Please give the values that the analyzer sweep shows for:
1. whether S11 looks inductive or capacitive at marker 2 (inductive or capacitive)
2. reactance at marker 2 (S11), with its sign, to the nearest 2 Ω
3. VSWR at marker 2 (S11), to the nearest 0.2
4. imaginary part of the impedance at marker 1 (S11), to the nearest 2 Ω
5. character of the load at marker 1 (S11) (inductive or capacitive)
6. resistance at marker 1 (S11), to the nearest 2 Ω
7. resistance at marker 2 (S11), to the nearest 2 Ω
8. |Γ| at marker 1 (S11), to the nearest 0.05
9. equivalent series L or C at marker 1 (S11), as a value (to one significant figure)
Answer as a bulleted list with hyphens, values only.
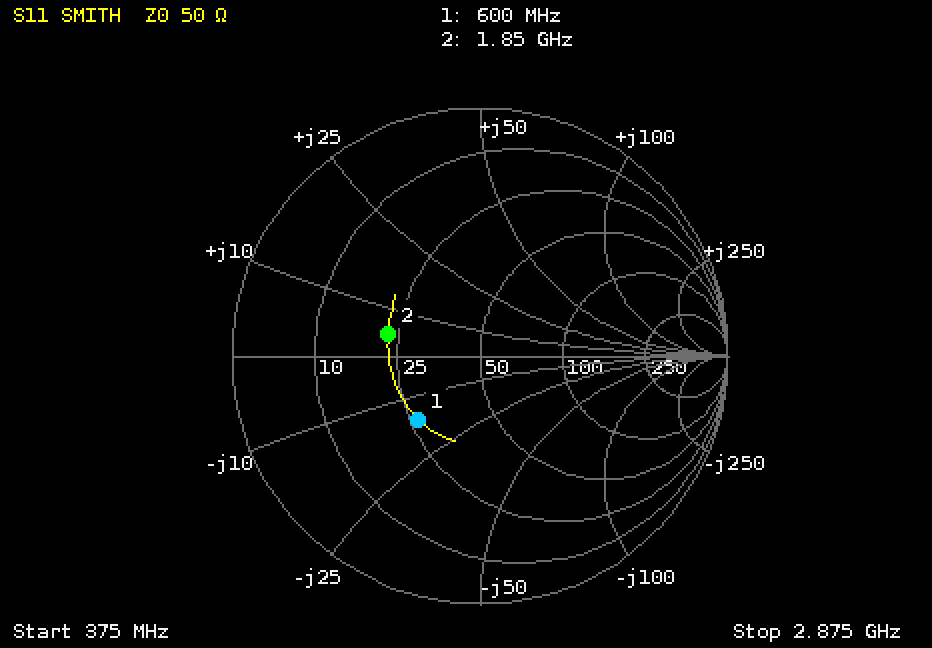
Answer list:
- inductive
- +4 Ω
- 2.2
- -16 Ω
- capacitive
- 26 Ω
- 22 Ω
- 0.35
- 20 pF
